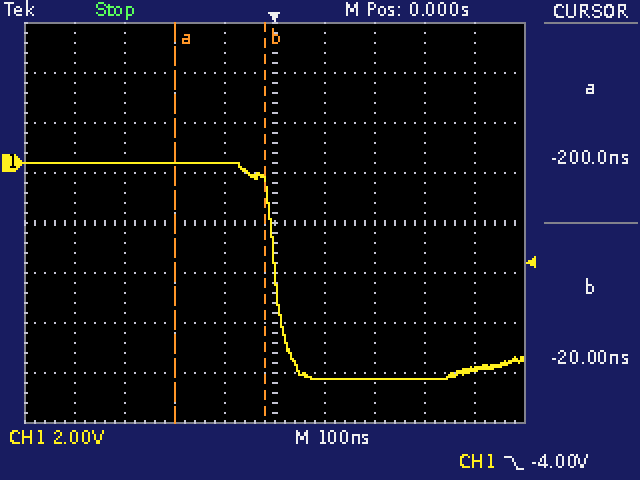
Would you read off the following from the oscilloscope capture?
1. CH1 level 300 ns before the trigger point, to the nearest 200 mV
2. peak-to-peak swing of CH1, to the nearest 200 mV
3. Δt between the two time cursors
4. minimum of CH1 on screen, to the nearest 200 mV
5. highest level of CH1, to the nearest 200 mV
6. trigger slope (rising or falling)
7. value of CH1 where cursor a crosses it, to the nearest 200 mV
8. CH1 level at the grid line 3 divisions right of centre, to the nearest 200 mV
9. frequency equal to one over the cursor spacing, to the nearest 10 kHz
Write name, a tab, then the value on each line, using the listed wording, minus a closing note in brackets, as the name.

CH1 level 300 ns before the trigger point, to the nearest 200 mV	0.0 V
peak-to-peak swing of CH1, to the nearest 200 mV	8.6 V
Δt between the two time cursors	180 ns
minimum of CH1 on screen, to the nearest 200 mV	-8.6 V
highest level of CH1, to the nearest 200 mV	0.0 V
trigger slope	falling
value of CH1 where cursor a crosses it, to the nearest 200 mV	0.0 V
CH1 level at the grid line 3 divisions right of centre, to the nearest 200 mV	-8.6 V
frequency equal to one over the cursor spacing, to the nearest 10 kHz	5.56 MHz
